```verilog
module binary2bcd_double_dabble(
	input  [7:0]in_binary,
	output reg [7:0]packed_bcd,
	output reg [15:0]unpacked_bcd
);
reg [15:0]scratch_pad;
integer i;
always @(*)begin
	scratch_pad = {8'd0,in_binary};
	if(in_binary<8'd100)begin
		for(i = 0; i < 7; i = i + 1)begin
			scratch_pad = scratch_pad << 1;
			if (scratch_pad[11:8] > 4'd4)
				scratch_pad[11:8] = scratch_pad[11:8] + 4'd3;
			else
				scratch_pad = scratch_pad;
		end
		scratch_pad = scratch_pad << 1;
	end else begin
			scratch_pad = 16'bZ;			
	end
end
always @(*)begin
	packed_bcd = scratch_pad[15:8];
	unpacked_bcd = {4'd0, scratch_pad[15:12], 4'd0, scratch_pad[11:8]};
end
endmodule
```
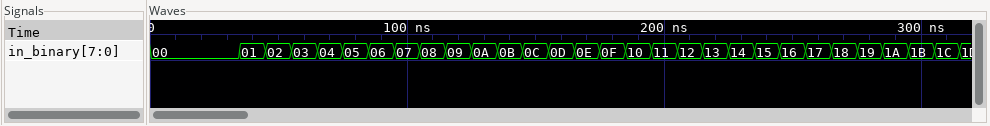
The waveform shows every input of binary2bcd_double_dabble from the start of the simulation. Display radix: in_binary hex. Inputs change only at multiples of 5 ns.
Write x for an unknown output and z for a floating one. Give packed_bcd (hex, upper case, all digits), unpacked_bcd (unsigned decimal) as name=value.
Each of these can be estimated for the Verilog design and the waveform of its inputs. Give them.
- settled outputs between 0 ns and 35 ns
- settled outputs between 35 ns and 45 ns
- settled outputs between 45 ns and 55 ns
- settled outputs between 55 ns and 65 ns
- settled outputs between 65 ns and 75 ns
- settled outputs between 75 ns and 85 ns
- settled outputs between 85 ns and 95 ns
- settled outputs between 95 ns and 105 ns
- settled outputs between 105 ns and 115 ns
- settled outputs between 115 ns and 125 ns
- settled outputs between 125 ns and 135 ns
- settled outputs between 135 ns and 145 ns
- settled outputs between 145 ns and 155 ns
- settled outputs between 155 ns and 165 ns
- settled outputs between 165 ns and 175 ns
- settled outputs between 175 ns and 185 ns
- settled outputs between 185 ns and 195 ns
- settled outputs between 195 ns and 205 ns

packed_bcd=00, unpacked_bcd=0
packed_bcd=01, unpacked_bcd=1
packed_bcd=02, unpacked_bcd=2
packed_bcd=03, unpacked_bcd=3
packed_bcd=04, unpacked_bcd=4
packed_bcd=05, unpacked_bcd=5
packed_bcd=06, unpacked_bcd=6
packed_bcd=07, unpacked_bcd=7
packed_bcd=08, unpacked_bcd=8
packed_bcd=09, unpacked_bcd=9
packed_bcd=10, unpacked_bcd=256
packed_bcd=11, unpacked_bcd=257
packed_bcd=12, unpacked_bcd=258
packed_bcd=13, unpacked_bcd=259
packed_bcd=14, unpacked_bcd=260
packed_bcd=15, unpacked_bcd=261
packed_bcd=16, unpacked_bcd=262
packed_bcd=17, unpacked_bcd=263
